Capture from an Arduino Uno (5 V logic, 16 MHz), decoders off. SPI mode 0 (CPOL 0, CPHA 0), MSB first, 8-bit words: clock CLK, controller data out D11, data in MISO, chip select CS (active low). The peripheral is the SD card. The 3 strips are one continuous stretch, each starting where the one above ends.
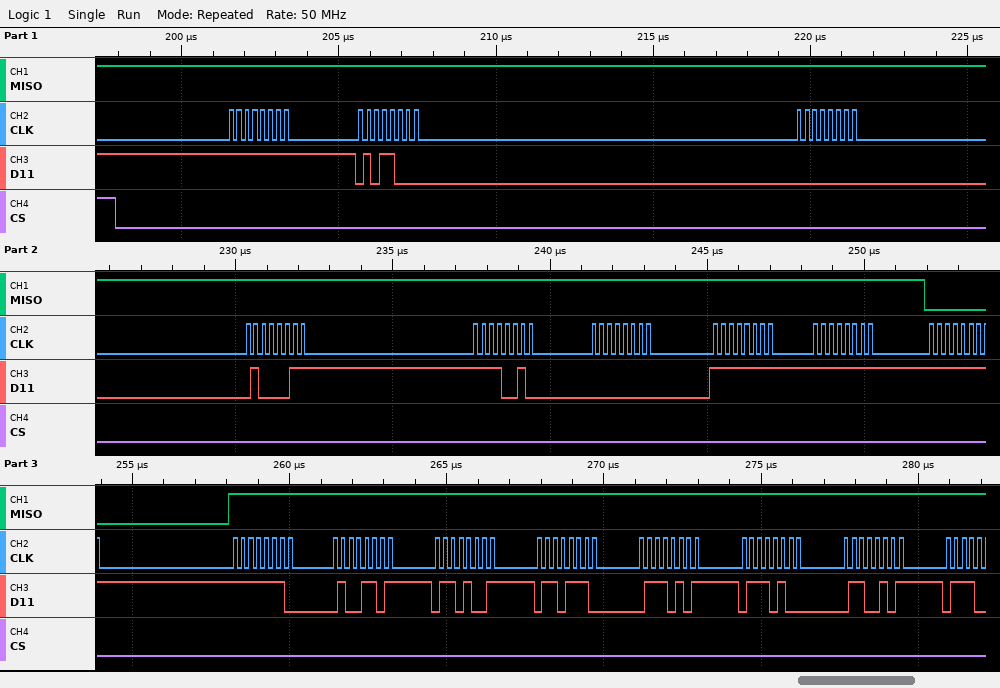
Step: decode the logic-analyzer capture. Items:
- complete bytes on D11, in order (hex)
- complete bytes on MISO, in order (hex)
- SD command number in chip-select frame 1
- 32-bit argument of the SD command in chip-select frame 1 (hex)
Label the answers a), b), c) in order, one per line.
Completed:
a) FF 58 00 43 F2 00 FF FF FF FE 4D 69 6E 75 74 65
b) FF FF FF FF FF FF FF FF 00 FF FF FF FF FF FF FF
c) CMD24
d) 0x0043F200
